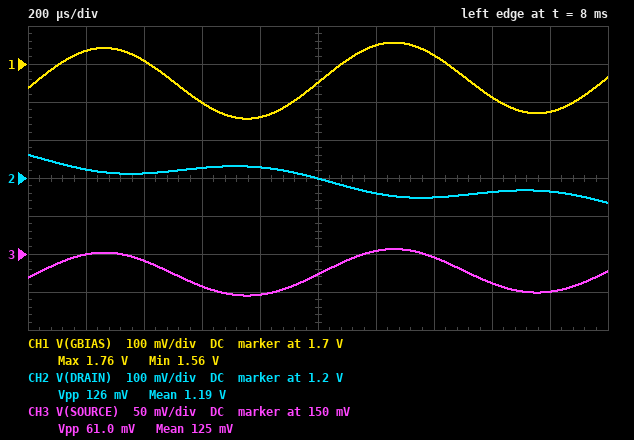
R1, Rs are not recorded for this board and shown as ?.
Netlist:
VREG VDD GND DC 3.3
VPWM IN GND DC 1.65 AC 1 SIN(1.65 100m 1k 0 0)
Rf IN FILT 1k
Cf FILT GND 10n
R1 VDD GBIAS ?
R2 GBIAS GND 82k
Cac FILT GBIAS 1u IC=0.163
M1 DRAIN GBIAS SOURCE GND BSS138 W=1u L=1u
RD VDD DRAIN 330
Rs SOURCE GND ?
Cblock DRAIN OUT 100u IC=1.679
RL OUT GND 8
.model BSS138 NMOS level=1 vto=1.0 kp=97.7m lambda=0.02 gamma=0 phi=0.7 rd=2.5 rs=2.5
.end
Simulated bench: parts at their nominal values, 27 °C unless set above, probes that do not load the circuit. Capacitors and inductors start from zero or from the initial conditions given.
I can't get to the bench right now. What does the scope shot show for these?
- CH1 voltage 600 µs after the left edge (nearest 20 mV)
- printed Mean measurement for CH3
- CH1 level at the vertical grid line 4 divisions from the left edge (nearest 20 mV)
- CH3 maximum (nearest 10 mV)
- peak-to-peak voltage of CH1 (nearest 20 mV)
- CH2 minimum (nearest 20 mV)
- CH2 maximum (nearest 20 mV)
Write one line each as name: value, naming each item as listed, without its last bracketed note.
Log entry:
CH1 voltage 600 µs after the left edge: 1.60 V
printed Mean measurement for CH3: 125 mV
CH1 level at the vertical grid line 4 divisions from the left edge: 1.56 V
CH3 maximum: 160 mV
peak-to-peak voltage of CH1: 200 mV
CH2 minimum: 1.14 V
CH2 maximum: 1.26 V
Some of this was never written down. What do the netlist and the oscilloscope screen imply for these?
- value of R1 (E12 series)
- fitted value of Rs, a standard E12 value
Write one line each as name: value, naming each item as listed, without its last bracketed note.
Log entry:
value of R1: 47 kΩ
fitted value of Rs, a standard E12 value: 10 Ω
